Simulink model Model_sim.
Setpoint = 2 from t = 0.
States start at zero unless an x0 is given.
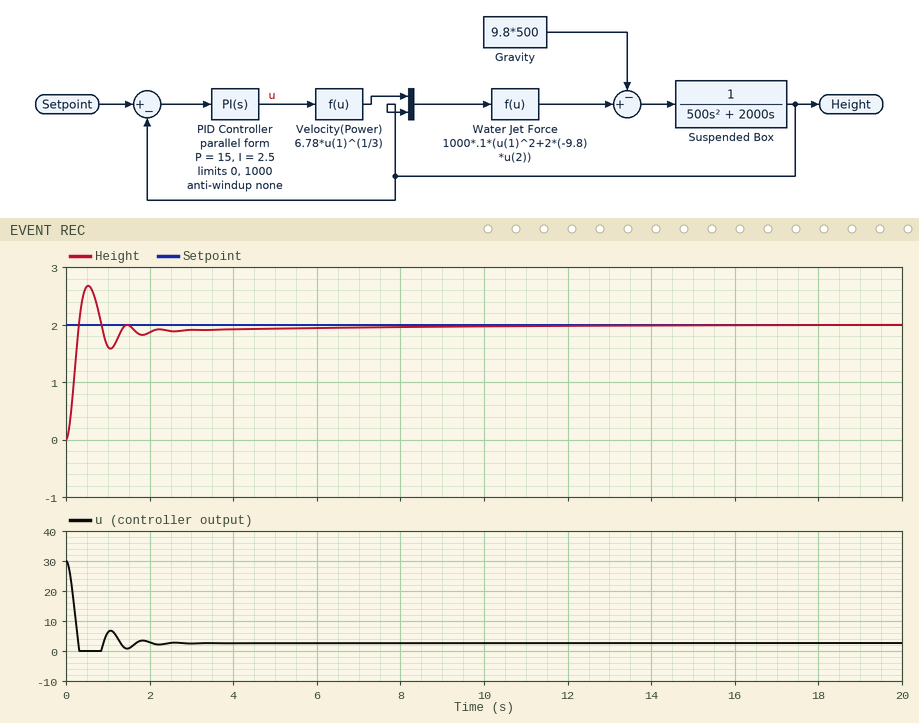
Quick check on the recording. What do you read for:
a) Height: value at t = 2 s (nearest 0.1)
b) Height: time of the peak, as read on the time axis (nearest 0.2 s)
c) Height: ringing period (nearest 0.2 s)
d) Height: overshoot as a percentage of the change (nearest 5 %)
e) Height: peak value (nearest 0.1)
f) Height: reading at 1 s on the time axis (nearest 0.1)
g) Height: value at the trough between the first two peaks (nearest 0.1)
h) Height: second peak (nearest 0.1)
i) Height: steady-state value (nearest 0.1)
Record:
1.9
0.6 s
1.0 s
35 %
2.7
1.6
1.6
2.0
2.0
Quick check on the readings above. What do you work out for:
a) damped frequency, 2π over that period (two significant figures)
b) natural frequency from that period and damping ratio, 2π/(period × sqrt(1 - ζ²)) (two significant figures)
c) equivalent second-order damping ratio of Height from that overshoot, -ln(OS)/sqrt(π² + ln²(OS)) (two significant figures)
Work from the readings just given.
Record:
6.3 rad/s
6.6 rad/s
0.32
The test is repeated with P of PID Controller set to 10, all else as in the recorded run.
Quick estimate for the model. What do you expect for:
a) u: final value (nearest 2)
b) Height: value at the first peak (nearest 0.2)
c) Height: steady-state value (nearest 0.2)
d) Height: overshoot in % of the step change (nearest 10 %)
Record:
2
2.4
2.0
20 %
